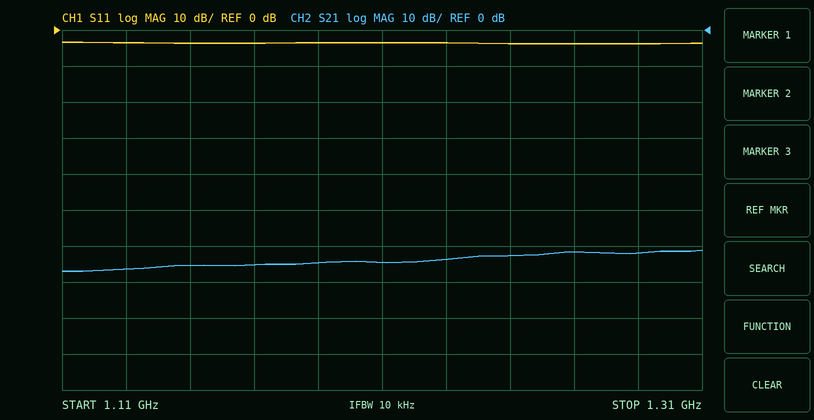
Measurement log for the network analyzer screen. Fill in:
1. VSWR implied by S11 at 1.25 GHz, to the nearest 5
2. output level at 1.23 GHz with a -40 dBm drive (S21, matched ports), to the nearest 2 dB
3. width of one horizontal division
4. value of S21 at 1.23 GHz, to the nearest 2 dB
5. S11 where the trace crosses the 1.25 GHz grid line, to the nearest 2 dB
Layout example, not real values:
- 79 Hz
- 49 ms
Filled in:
- 5
- -104 dBm
- 20 MHz
- -64 dB
- -4 dB
